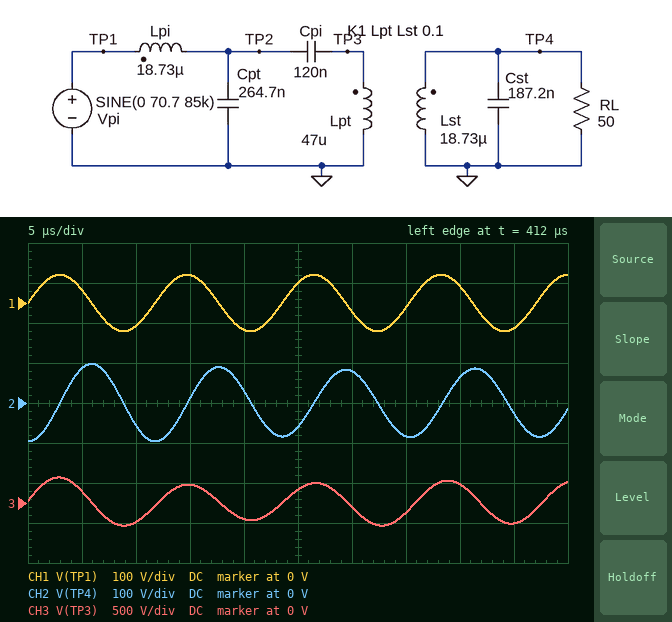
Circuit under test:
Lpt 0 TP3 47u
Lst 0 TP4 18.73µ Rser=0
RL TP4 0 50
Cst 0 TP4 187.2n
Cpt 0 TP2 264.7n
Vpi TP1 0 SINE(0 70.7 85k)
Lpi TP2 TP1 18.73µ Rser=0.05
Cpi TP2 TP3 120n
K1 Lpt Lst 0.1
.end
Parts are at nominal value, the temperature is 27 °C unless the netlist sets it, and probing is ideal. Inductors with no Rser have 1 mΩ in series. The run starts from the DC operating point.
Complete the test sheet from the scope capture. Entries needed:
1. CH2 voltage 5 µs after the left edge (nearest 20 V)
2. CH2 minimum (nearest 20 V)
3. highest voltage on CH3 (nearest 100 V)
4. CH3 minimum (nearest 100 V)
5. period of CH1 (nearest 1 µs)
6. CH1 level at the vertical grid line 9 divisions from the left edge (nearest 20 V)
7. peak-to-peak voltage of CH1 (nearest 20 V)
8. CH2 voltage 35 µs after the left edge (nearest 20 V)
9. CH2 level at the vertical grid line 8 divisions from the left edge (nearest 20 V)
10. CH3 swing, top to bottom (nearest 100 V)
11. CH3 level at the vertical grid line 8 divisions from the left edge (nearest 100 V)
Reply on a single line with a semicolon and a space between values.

80 V; -100 V; 300 V; -300 V; 12 µs; -60 V; 140 V; -80 V; 60 V; 600 V; 200 V
